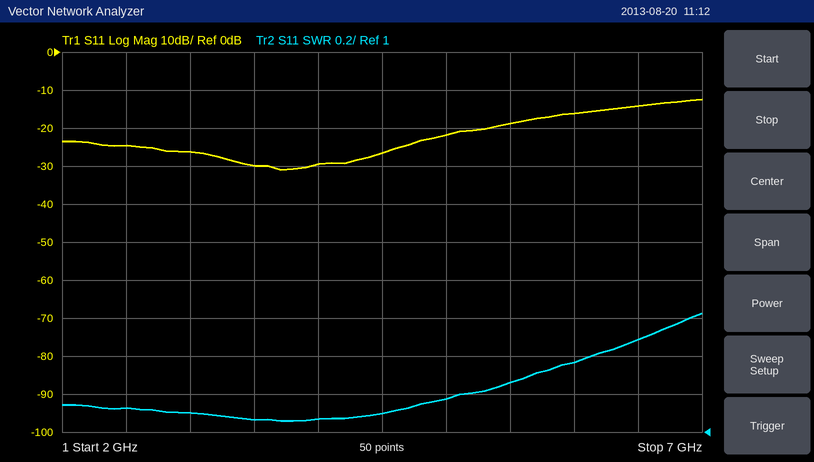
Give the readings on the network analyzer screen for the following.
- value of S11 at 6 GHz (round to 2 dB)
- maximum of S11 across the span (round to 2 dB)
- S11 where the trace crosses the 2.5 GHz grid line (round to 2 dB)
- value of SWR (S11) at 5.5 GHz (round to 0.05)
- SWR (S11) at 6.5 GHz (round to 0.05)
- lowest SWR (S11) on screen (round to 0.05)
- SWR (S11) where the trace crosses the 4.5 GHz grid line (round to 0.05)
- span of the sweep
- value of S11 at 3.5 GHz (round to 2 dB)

-16 dB
-12 dB
-24 dB
1.25
1.50
1.05
1.10
5 GHz
-30 dB
